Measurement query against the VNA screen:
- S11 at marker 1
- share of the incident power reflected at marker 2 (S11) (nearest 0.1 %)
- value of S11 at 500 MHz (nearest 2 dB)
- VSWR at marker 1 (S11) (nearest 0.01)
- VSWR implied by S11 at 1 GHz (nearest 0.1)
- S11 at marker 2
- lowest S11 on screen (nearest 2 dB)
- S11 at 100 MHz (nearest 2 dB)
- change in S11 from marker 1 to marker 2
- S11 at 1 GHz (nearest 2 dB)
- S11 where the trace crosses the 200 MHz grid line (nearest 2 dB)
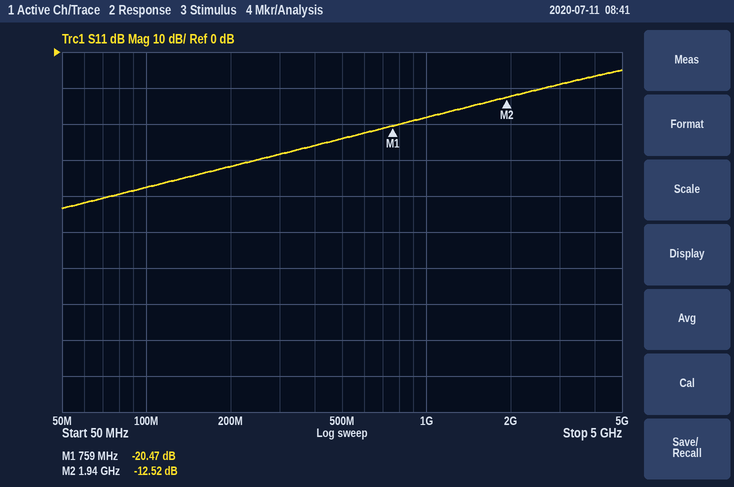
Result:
-20.47 dB
5.6 %
-24 dB
1.21
1.3
-12.52 dB
-44 dB
-38 dB
7.95 dB
-18 dB
-32 dB
